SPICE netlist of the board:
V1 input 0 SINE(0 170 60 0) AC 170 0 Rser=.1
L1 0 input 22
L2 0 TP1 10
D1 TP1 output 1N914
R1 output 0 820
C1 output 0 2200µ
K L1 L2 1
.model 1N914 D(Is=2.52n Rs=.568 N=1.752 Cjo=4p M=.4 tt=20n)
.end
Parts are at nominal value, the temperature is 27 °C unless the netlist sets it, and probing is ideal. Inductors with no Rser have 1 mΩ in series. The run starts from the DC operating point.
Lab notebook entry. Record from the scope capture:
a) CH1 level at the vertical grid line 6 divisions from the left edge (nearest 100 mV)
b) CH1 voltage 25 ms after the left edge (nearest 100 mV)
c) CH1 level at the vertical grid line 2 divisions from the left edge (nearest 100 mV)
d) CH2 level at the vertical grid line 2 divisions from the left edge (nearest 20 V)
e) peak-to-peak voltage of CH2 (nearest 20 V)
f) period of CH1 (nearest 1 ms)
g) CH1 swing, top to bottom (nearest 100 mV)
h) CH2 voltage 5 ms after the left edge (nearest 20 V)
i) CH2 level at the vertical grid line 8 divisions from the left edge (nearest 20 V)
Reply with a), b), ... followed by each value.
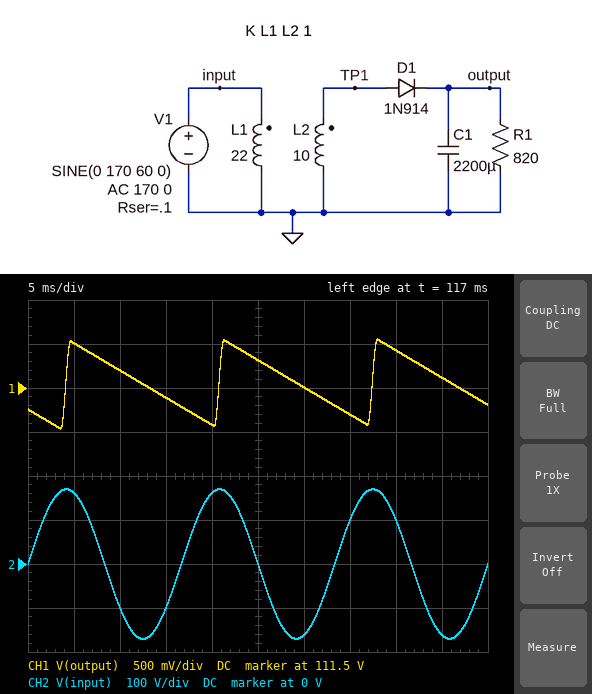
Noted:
a) 111.5 V
b) 111.8 V
c) 111.7 V
d) -100 V
e) 340 V
f) 17 ms
g) 1.0 V
h) 160 V
i) 100 V
